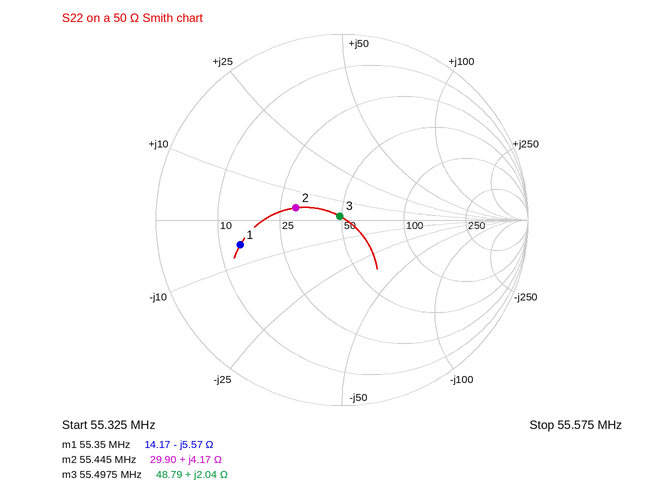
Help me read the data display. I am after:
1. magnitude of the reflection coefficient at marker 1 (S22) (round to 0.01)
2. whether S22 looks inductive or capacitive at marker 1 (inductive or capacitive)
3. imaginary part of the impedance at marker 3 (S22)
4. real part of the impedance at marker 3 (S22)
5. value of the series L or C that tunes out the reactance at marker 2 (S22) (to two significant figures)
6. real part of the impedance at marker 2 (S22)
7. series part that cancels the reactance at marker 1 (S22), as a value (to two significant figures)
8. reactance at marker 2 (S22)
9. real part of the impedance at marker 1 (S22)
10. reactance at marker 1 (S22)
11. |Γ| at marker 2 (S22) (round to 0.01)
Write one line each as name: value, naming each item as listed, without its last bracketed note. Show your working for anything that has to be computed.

magnitude of the reflection coefficient at marker 1 (S22): 0.56
whether S22 looks inductive or capacitive at marker 1: capacitive
imaginary part of the impedance at marker 3: +2.04 Ω
real part of the impedance at marker 3: 48.79 Ω
value of the series L or C that tunes out the reactance at marker 2 (S22): C = 1/(2π × 55.445 MHz × 4.17 Ω) ≈ 688 pF, so 690 pF to two significant figures
real part of the impedance at marker 2: 29.90 Ω
series part that cancels the reactance at marker 1 (S22), as a value: L = 5.57 Ω/(2π × 55.35 MHz) ≈ 16 nH
reactance at marker 2: +4.17 Ω
real part of the impedance at marker 1: 14.17 Ω
reactance at marker 1: -5.57 Ω
|Γ| at marker 2 (S22): 0.26
